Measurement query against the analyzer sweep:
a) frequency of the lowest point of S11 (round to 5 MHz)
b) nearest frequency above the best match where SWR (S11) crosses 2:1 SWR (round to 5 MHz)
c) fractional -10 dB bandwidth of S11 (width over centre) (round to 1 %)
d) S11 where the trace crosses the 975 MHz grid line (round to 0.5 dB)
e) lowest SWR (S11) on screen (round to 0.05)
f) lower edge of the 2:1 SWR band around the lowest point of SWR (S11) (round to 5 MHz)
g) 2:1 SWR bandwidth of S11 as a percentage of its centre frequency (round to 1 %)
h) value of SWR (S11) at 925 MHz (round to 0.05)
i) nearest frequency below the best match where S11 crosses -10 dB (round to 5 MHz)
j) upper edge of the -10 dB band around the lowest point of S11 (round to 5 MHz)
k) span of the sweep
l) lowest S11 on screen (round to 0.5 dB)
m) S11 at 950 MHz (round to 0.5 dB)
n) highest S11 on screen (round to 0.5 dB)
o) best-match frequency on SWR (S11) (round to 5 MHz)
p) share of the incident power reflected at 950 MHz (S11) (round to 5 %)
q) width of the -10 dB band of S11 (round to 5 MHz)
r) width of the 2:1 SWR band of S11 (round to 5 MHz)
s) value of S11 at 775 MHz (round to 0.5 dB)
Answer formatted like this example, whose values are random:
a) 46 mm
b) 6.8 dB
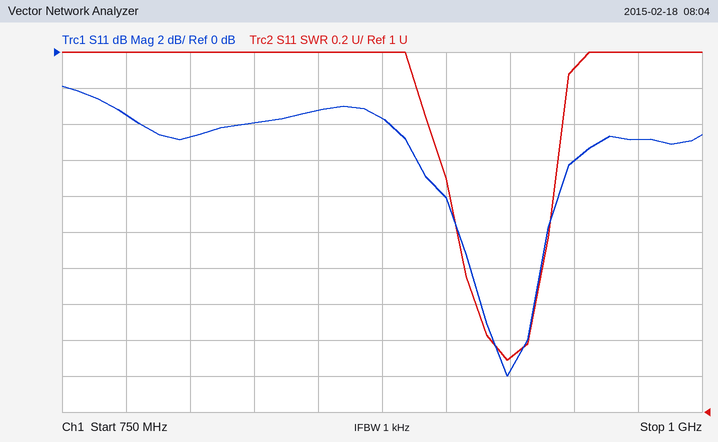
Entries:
a) 925 MHz
b) 940 MHz
c) 4 %
d) -5.0 dB
e) 1.30
f) 905 MHz
g) 4 %
h) 1.30
i) 905 MHz
j) 940 MHz
k) 250 MHz
l) -18.0 dB
m) -6.0 dB
n) -2.0 dB
o) 925 MHz
p) 25 %
q) 35 MHz
r) 35 MHz
s) -3.5 dB
